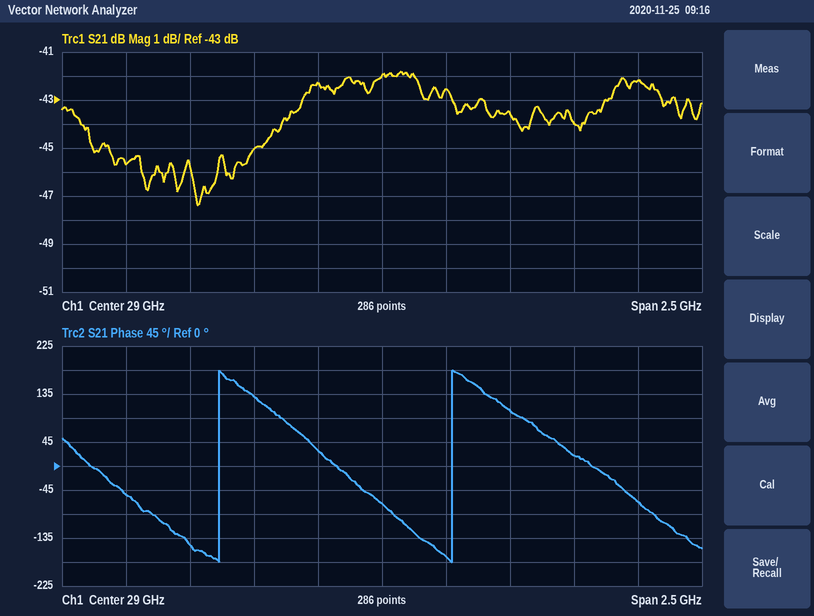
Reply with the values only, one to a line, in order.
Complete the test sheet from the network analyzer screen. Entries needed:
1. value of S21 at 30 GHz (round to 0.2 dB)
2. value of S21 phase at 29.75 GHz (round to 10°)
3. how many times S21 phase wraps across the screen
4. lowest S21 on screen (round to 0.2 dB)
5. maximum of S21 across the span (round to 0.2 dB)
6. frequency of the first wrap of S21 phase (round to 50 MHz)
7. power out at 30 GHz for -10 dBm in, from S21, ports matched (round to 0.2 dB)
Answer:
-42.2 dB
20°
2
-47.4 dB
-41.8 dB
28.35 GHz
-52.2 dBm
